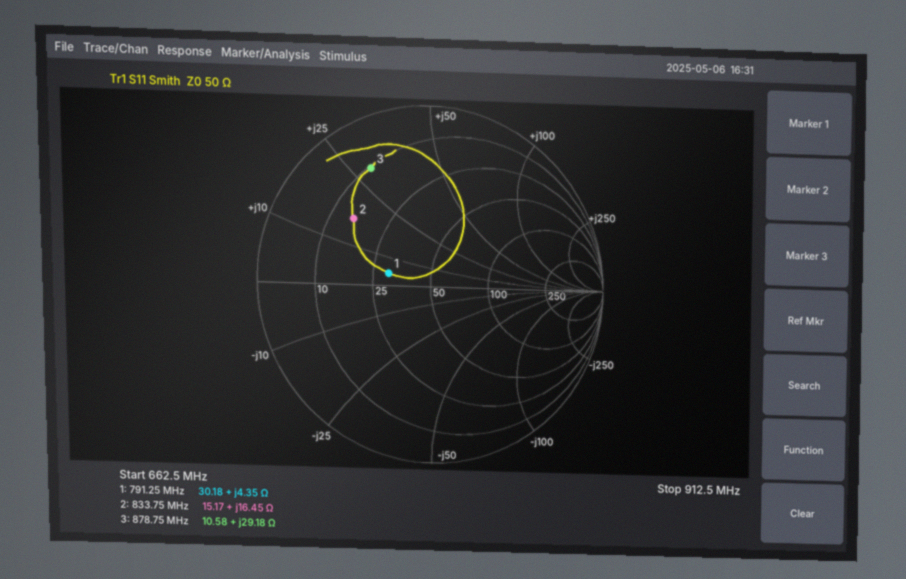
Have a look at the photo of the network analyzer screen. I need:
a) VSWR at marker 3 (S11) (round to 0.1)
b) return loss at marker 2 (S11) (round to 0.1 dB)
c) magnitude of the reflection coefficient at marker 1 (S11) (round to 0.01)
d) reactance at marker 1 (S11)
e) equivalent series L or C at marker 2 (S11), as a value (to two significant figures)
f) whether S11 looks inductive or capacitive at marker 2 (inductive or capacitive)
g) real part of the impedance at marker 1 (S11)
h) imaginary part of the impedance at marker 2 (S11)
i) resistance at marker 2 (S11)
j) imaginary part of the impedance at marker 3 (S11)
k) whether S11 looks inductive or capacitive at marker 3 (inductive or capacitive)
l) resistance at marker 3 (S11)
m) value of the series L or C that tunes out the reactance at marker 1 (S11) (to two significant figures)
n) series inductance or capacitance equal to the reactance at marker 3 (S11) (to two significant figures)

6.4
4.8 dB
0.25
+4.35 Ω
3.1 nH
inductive
30.18 Ω
+16.45 Ω
15.17 Ω
+29.18 Ω
inductive
10.58 Ω
46 pF
5.3 nH
